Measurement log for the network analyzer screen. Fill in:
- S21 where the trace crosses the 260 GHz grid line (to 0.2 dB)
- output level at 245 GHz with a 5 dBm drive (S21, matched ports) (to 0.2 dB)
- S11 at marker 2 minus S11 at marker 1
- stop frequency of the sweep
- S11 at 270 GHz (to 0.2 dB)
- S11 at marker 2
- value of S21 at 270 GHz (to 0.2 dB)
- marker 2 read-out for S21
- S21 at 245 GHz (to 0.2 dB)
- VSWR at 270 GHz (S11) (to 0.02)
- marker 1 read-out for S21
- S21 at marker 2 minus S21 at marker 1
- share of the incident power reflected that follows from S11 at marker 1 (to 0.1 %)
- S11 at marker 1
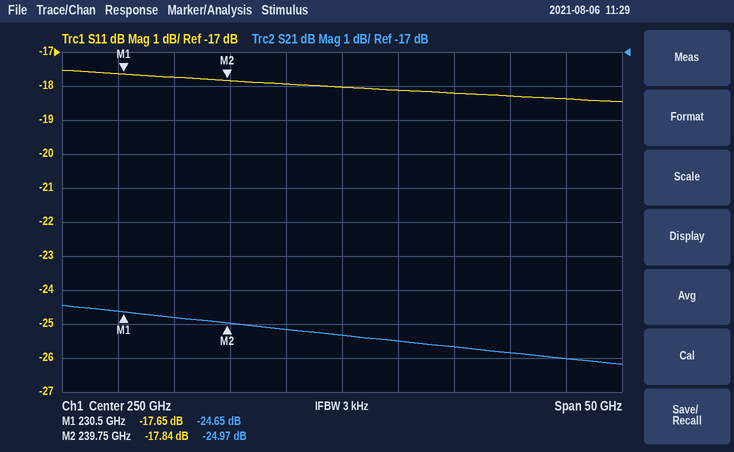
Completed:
-25.6 dB
-20.2 dBm
-0.19 dB
275 GHz
-18.4 dB
-17.84 dB
-26.0 dB
-24.97 dB
-25.2 dB
1.28
-24.65 dB
-0.32 dB
1.7 %
-17.65 dB
